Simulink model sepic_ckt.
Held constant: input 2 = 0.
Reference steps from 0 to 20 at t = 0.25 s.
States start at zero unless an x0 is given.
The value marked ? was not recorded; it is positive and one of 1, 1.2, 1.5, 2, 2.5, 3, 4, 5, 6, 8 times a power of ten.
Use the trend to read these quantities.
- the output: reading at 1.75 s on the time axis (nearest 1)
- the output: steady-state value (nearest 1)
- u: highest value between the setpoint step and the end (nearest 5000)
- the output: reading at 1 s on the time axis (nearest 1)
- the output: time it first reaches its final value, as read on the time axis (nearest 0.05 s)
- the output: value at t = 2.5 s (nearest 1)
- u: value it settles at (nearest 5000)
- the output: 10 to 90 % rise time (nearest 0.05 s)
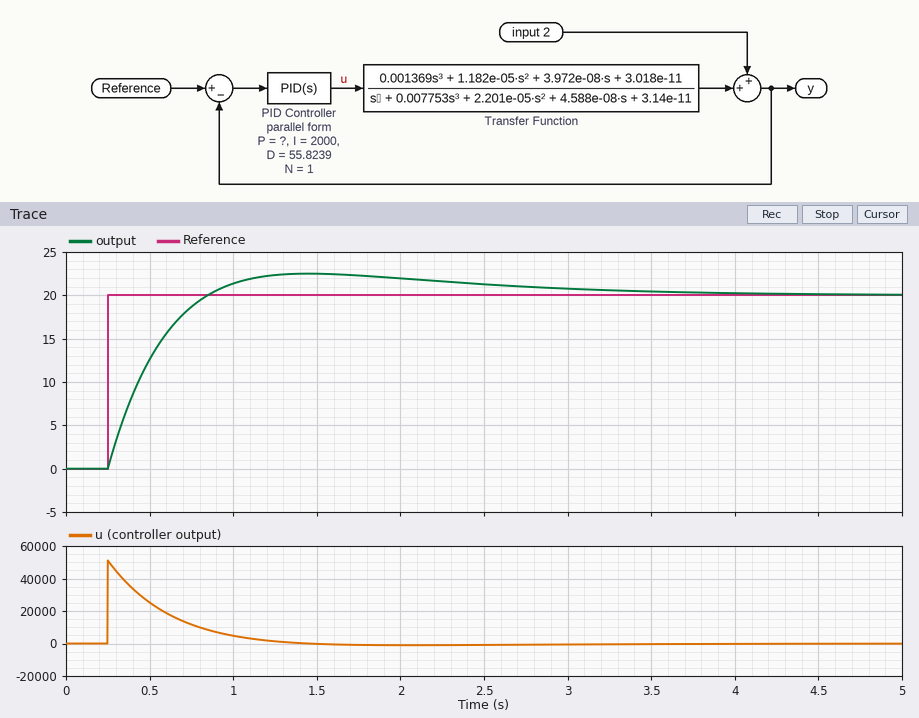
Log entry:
22
20
50000
21
0.85 s
21
0
0.45 s
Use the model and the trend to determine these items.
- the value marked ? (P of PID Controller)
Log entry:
2500
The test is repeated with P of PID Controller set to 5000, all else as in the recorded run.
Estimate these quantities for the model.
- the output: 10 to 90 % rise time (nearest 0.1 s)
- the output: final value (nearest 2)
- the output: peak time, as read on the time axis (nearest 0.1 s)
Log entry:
0.3 s
20
1.2 s
